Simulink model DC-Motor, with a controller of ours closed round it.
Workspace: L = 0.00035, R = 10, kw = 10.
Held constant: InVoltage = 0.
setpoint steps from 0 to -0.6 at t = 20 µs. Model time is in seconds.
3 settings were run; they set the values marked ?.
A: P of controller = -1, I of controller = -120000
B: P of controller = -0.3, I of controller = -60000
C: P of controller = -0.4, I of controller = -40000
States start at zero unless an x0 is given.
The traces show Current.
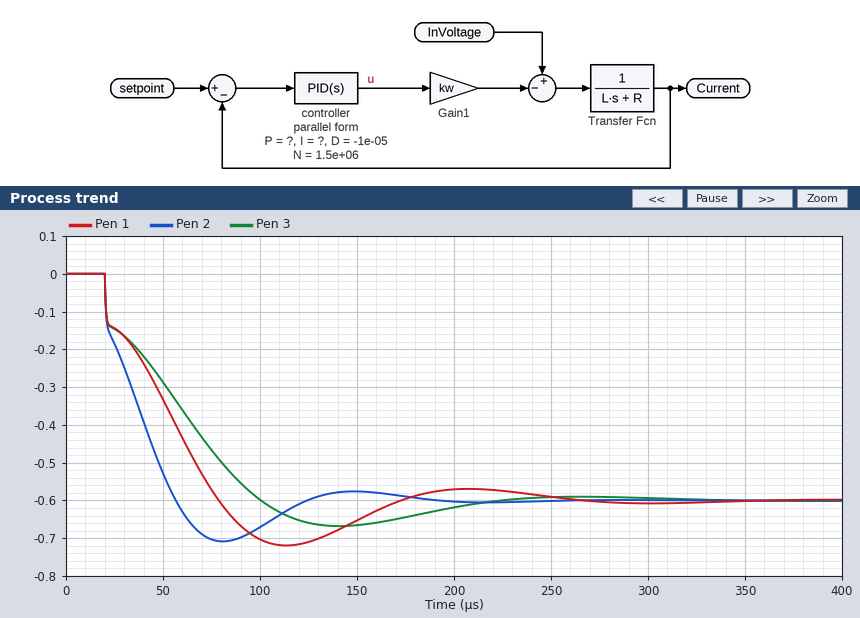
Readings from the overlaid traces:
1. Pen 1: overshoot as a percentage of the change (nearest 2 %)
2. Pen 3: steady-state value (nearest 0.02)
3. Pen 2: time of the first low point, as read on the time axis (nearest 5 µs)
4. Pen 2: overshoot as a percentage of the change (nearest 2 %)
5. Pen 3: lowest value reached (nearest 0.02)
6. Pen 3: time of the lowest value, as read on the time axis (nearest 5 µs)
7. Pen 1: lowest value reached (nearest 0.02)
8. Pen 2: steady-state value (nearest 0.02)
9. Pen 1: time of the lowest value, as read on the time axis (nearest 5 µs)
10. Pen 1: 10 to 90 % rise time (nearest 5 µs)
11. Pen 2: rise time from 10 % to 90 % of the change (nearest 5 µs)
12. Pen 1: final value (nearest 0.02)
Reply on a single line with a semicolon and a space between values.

20 %; -0.60; 80 µs; 18 %; -0.66; 140 µs; -0.72; -0.60; 115 µs; 50 µs; 30 µs; -0.60
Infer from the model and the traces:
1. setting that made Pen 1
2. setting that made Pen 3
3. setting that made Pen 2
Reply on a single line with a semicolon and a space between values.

B; C; A
